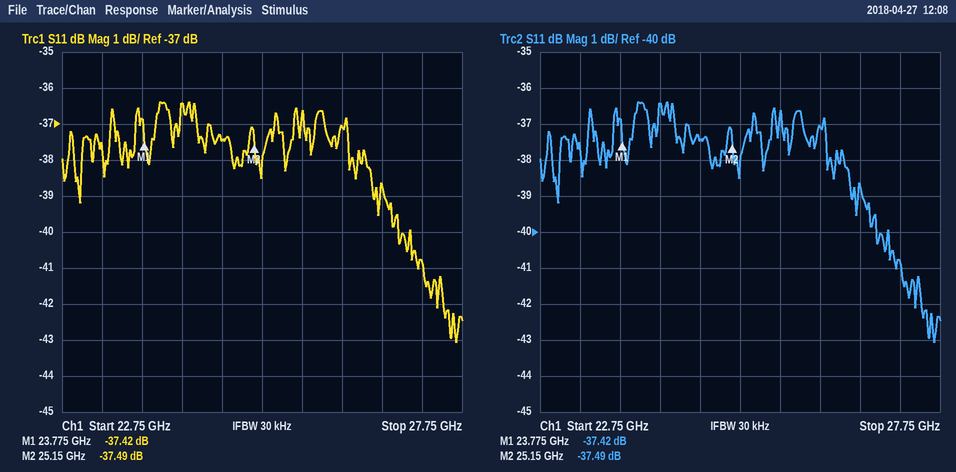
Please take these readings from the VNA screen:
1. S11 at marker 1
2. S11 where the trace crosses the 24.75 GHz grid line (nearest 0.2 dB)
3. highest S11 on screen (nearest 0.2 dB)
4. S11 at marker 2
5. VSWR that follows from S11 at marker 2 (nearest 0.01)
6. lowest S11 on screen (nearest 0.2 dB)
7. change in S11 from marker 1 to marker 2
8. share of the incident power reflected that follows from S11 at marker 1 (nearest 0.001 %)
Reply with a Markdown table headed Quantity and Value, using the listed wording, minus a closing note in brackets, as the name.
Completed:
| Quantity | Value |
|---|---|
| S11 at marker 1 | -37.42 dB |
| S11 where the trace crosses the 24.75 GHz grid line | -37.4 dB |
| highest S11 on screen | -36.4 dB |
| S11 at marker 2 | -37.49 dB |
| VSWR that follows from S11 at marker 2 | 1.03 |
| lowest S11 on screen | -43.0 dB |
| change in S11 from marker 1 to marker 2 | -0.07 dB |
| share of the incident power reflected that follows from S11 at marker 1 | 0.018 % |
